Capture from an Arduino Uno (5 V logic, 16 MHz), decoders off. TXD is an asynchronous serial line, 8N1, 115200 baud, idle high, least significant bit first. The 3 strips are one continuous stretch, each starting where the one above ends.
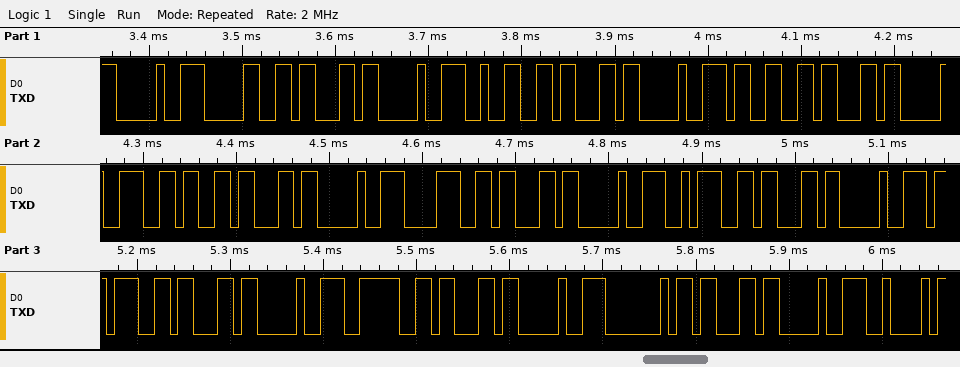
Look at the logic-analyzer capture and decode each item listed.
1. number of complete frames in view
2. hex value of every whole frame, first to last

29
0x90 0x30 0x63 0x90 0x32 0x63 0x90 0x33 0x63 0x90 0x36 0x63 0x90 0x38 0x63 0x90 0x3A 0x63 0x90 0x3B 0x63 0x90 0x3E 0x63 0x90 0x40 0x63 0x90 0x42
